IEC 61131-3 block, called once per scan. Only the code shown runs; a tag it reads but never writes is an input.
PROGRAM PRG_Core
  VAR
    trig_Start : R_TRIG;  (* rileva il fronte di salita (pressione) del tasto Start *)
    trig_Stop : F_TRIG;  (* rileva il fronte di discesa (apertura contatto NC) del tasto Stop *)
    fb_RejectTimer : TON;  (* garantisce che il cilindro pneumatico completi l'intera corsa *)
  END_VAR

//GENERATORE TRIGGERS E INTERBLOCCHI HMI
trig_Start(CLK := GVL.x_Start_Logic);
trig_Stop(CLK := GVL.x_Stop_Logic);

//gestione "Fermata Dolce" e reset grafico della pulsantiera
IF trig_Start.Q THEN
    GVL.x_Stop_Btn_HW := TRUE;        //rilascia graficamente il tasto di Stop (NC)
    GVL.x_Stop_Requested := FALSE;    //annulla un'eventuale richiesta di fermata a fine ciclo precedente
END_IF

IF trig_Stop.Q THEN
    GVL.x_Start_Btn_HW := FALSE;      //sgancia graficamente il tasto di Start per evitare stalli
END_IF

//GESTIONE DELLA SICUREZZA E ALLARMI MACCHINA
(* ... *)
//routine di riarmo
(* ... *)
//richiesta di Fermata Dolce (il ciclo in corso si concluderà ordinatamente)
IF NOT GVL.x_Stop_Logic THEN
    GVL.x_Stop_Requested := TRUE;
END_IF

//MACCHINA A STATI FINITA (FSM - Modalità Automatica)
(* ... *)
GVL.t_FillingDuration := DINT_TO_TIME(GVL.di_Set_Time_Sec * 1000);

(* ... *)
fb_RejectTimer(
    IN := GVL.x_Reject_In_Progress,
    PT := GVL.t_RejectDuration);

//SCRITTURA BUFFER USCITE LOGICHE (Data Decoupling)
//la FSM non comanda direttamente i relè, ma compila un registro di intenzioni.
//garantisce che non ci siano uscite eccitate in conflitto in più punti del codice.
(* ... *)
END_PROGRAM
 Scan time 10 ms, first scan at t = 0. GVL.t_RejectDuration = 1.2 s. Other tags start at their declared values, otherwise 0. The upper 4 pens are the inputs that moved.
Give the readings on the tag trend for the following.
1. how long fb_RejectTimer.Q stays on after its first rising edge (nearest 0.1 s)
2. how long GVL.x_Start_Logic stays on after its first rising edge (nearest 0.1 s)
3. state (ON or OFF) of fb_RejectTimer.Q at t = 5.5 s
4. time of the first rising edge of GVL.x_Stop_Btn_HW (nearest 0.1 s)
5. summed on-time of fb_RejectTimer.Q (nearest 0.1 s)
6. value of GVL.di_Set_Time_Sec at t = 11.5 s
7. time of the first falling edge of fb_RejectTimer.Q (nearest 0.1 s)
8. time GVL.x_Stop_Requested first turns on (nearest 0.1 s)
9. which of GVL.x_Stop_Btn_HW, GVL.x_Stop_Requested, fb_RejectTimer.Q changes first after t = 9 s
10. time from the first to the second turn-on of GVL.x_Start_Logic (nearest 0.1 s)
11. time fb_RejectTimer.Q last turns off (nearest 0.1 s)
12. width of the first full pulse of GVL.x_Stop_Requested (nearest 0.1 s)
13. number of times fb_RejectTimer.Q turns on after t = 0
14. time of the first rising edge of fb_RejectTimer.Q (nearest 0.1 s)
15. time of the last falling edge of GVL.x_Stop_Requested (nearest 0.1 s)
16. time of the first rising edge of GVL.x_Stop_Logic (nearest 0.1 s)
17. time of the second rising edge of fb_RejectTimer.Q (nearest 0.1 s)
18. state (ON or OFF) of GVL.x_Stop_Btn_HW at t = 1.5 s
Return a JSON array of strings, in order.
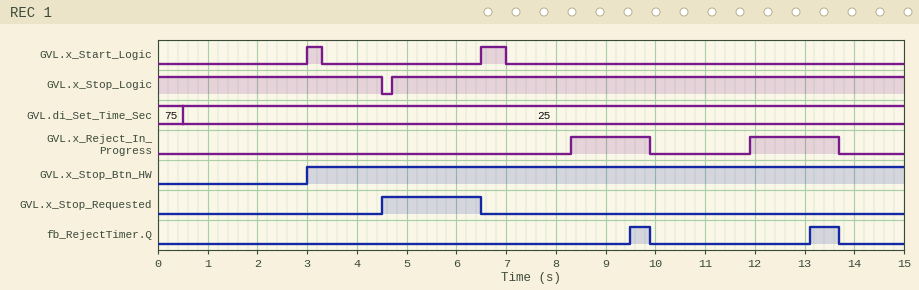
["0.4 s", "0.3 s", "OFF", "3.0 s", "1.0 s", "25", "9.9 s", "4.5 s", "fb_RejectTimer.Q", "3.5 s", "13.7 s", "2.0 s", "2", "9.5 s", "6.5 s", "4.7 s", "13.1 s", "OFF"]
